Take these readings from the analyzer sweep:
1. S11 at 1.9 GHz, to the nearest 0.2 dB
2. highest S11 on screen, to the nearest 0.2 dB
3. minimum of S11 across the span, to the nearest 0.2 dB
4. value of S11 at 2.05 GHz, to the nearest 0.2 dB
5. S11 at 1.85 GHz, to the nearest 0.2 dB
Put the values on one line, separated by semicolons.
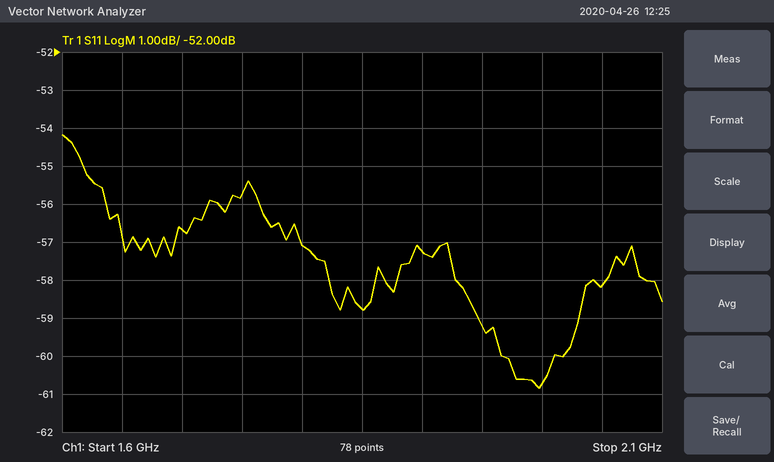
-57.2 dB; -54.2 dB; -60.8 dB; -58.2 dB; -58.8 dB
